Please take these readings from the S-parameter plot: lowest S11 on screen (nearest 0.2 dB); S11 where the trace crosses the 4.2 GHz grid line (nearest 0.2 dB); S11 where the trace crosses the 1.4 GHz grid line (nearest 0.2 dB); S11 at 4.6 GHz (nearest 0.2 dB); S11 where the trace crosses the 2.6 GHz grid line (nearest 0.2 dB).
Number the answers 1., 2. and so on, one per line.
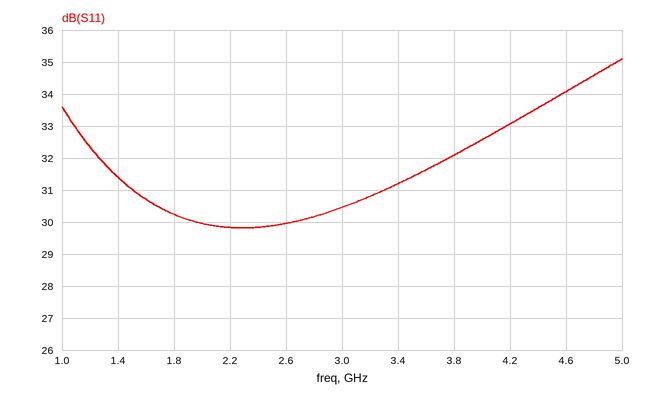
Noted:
1. 29.8 dB
2. 33.0 dB
3. 31.4 dB
4. 34.0 dB
5. 30.0 dB
